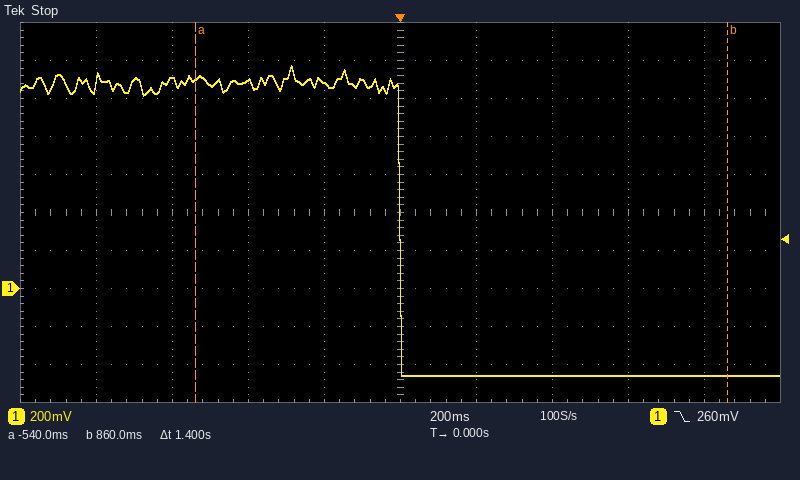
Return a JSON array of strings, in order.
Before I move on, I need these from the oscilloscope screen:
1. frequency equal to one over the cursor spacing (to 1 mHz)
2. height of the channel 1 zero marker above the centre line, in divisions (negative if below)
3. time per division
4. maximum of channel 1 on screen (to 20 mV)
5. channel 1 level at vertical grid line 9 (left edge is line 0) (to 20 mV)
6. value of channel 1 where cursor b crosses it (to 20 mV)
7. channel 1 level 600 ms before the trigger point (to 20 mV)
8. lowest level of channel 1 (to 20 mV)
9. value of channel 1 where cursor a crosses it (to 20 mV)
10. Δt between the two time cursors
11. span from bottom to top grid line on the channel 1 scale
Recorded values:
["714 mHz", "-2.0 div", "200 ms", "1.18 V", "-460 mV", "-460 mV", "1.10 V", "-460 mV", "1.10 V", "1.4 s", "2 V"]
